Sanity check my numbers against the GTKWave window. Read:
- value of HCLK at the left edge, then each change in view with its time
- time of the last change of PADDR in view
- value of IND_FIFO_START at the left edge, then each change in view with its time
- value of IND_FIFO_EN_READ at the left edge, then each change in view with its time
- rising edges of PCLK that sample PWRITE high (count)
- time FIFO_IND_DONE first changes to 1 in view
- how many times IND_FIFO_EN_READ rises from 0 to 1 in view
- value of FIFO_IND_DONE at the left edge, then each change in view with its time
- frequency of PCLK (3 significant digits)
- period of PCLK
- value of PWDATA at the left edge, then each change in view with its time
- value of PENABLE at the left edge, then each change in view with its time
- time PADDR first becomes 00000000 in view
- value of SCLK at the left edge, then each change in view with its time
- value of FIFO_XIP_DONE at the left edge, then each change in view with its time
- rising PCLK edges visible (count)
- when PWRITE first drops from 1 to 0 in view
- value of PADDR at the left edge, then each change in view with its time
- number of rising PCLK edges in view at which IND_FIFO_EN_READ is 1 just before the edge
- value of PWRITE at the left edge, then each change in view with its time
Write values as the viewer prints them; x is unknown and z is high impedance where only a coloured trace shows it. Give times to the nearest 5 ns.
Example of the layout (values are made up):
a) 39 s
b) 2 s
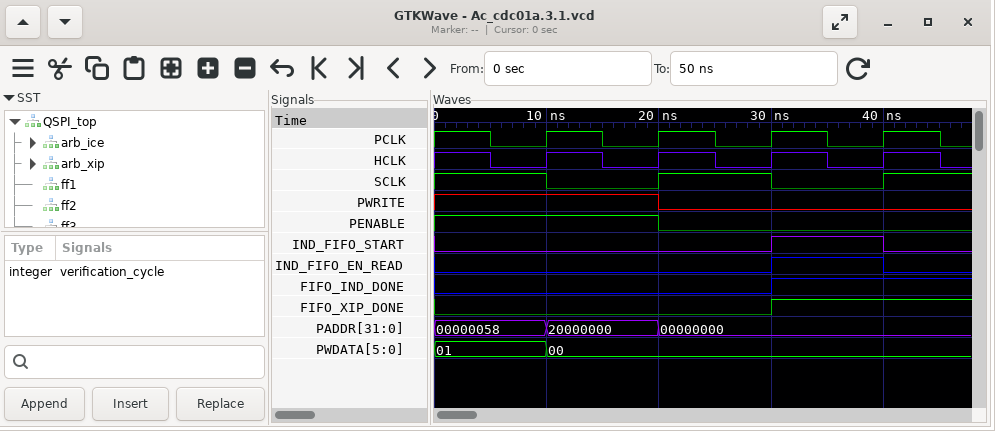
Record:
a) 1, 0 at 5 ns, 1 at 10 ns, 0 at 15 ns, 1 at 20 ns, 0 at 25 ns, 1 at 30 ns, 0 at 35 ns, 1 at 40 ns, 0 at 45 ns
b) 20 ns
c) 0, 1 at 30 ns, 0 at 40 ns
d) 0, 1 at 30 ns, 0 at 40 ns
e) 2
f) 30 ns
g) 1
h) 0, 1 at 30 ns
i) 100 MHz
j) 10 ns
k) 01, 00 at 10 ns
l) 1, 0 at 20 ns
m) 20 ns
n) 1, 0 at 10 ns, 1 at 20 ns, 0 at 30 ns, 1 at 40 ns
o) 0, 1 at 30 ns
p) 4
q) 20 ns
r) 00000058, 20000000 at 10 ns, 00000000 at 20 ns
s) 1
t) 1, 0 at 20 ns
